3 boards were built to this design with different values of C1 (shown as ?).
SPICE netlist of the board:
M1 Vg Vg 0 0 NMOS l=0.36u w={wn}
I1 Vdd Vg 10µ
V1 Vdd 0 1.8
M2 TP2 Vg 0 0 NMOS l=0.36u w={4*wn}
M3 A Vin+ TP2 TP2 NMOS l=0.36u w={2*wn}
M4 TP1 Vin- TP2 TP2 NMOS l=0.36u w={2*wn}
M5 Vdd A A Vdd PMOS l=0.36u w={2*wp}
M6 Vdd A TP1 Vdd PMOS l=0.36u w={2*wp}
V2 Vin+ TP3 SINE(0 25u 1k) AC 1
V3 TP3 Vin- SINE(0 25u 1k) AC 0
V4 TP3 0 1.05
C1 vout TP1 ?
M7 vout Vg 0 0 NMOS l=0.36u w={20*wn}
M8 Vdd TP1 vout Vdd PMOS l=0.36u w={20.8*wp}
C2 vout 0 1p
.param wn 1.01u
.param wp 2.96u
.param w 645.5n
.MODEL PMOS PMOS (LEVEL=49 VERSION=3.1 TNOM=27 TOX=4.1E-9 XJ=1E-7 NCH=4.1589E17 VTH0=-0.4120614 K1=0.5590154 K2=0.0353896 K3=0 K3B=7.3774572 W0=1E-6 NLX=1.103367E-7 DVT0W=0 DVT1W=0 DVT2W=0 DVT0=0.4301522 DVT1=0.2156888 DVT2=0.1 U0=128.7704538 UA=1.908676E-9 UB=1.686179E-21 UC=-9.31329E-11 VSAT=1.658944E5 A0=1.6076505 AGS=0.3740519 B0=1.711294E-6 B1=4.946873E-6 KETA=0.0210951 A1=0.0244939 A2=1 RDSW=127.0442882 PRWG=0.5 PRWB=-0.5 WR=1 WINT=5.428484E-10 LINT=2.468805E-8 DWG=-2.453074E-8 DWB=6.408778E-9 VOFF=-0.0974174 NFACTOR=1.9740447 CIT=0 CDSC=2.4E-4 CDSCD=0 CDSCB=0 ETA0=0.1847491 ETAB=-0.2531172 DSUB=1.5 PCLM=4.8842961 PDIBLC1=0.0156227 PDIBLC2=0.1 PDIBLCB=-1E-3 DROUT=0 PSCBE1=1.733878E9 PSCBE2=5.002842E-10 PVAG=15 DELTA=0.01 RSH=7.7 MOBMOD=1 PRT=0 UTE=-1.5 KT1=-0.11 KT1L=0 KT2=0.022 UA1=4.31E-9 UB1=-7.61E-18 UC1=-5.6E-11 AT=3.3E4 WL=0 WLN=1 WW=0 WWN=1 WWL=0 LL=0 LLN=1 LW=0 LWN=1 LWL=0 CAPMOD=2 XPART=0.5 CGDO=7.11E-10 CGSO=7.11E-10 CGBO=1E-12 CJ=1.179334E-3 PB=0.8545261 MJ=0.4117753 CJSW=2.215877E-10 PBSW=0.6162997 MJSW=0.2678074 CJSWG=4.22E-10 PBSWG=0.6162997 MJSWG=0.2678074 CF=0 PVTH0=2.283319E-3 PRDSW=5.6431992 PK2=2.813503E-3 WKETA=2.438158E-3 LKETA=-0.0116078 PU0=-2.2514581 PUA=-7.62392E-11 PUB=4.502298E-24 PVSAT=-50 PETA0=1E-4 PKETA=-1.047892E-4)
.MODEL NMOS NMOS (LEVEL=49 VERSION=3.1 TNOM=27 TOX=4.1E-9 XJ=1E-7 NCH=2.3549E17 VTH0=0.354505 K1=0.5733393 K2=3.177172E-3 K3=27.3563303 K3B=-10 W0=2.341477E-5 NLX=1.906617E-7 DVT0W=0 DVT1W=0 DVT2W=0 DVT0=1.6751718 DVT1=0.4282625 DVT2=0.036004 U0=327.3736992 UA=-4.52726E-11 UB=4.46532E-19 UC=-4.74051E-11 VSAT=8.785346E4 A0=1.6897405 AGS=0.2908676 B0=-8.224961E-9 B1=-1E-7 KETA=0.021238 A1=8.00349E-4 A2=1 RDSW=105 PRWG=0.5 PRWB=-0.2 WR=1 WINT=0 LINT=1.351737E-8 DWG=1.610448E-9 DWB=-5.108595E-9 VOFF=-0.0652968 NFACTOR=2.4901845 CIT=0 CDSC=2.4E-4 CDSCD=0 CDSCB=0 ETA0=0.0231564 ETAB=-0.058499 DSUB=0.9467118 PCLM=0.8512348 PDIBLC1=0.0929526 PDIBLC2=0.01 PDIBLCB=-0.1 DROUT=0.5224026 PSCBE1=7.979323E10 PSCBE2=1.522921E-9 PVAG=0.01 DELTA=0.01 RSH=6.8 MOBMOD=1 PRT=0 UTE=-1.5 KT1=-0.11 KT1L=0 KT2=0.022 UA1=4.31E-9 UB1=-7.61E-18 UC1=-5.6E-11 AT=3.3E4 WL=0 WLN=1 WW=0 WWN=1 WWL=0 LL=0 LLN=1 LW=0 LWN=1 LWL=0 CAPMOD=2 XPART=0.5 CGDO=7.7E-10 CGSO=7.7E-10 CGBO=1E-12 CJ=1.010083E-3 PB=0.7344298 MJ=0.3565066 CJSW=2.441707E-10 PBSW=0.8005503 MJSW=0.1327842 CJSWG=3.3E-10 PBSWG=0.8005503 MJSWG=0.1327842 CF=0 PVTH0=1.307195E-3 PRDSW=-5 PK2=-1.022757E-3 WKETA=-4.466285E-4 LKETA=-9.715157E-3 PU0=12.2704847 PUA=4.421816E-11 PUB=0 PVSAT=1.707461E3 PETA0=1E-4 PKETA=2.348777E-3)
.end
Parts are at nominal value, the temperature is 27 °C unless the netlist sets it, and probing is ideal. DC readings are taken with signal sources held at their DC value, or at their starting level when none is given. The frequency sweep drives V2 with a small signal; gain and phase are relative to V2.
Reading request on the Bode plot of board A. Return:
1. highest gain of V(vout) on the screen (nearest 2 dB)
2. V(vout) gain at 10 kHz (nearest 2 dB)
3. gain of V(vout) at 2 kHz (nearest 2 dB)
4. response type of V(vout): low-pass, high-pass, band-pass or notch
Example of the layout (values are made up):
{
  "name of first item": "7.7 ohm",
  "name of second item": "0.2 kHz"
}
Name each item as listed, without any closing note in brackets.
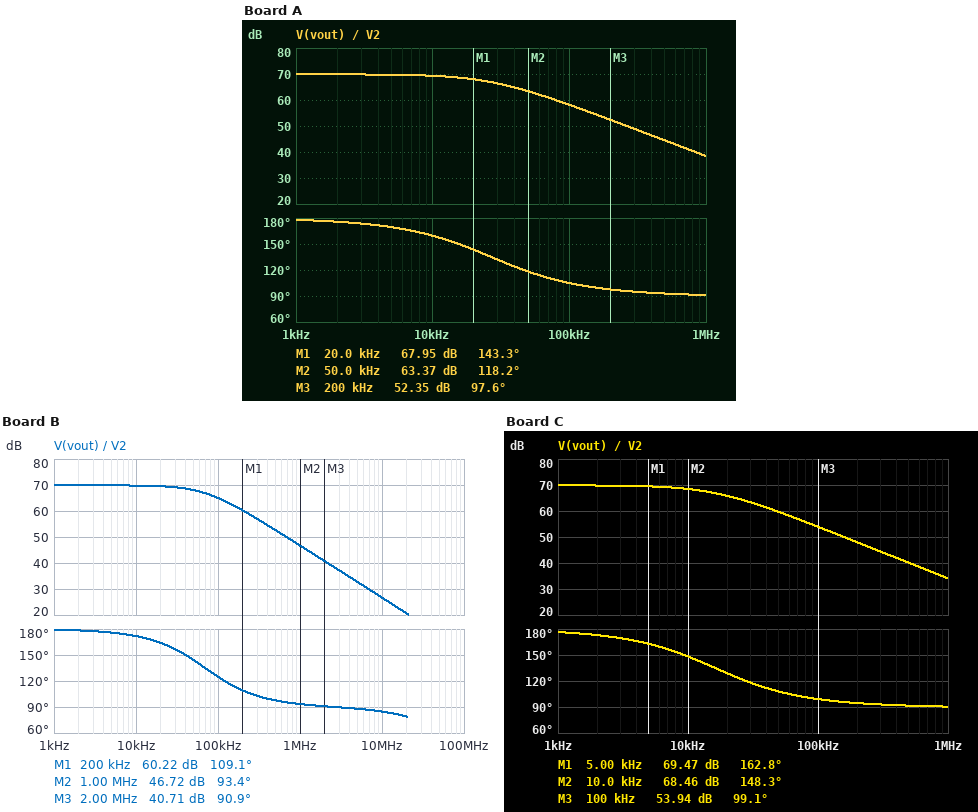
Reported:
{
  "highest gain of V(vout) on the screen": "70 dB",
  "V(vout) gain at 10 kHz": "70 dB",
  "gain of V(vout) at 2 kHz": "70 dB",
  "response type of V(vout): low-pass, high-pass, band-pass or notch": "low-pass"
}
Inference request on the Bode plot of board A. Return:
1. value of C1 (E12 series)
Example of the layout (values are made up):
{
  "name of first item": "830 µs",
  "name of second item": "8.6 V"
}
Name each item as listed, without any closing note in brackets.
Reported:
{
  "value of C1": "390 fF"
}
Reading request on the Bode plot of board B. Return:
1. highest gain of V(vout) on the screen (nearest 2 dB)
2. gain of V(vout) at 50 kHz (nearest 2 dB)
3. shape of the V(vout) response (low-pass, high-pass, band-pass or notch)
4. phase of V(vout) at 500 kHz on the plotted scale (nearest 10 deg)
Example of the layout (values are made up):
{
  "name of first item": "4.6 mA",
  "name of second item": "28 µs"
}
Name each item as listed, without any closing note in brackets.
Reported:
{
  "highest gain of V(vout) on the screen": "70 dB",
  "gain of V(vout) at 50 kHz": "68 dB",
  "shape of the V(vout) response": "low-pass",
  "phase of V(vout) at 500 kHz on the plotted scale": "100 deg"
}
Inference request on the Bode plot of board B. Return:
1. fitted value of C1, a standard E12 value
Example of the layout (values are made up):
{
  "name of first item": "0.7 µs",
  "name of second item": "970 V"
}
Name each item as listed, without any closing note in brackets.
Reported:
{
  "fitted value of C1, a standard E12 value": "120 fF"
}
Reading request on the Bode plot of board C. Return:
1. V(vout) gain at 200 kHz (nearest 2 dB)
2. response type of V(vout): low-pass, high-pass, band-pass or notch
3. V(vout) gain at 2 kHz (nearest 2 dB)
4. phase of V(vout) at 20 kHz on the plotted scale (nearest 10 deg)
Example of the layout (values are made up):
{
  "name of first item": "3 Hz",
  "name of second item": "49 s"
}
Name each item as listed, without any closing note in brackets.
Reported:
{
  "V(vout) gain at 200 kHz": "48 dB",
  "response type of V(vout): low-pass, high-pass, band-pass or notch": "low-pass",
  "V(vout) gain at 2 kHz": "70 dB",
  "phase of V(vout) at 20 kHz on the plotted scale": "130 deg"
}
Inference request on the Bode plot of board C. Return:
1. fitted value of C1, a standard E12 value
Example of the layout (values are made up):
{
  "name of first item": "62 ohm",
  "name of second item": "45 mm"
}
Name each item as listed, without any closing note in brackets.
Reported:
{
  "fitted value of C1, a standard E12 value": "680 fF"
}
